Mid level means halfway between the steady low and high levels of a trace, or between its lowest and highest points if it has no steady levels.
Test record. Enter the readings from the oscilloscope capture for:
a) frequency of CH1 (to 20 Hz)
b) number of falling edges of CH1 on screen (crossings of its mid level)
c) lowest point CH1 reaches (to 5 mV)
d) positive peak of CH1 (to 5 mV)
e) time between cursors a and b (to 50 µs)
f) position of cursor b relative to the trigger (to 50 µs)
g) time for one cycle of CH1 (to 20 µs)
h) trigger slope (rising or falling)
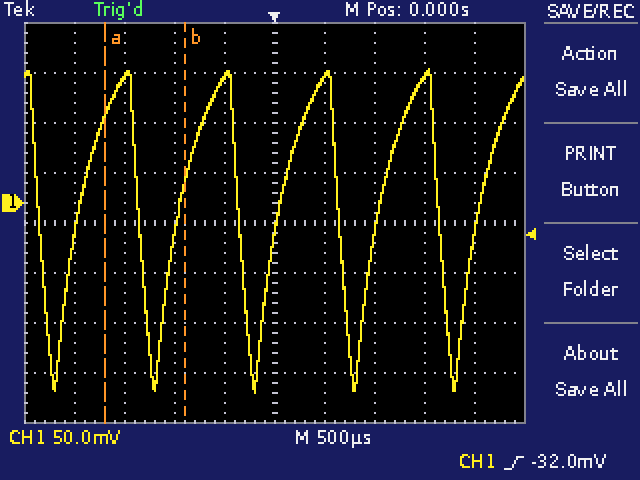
1.00 kHz
5
-190 mV
135 mV
800 µs
-900 µs
1.00 ms
rising
